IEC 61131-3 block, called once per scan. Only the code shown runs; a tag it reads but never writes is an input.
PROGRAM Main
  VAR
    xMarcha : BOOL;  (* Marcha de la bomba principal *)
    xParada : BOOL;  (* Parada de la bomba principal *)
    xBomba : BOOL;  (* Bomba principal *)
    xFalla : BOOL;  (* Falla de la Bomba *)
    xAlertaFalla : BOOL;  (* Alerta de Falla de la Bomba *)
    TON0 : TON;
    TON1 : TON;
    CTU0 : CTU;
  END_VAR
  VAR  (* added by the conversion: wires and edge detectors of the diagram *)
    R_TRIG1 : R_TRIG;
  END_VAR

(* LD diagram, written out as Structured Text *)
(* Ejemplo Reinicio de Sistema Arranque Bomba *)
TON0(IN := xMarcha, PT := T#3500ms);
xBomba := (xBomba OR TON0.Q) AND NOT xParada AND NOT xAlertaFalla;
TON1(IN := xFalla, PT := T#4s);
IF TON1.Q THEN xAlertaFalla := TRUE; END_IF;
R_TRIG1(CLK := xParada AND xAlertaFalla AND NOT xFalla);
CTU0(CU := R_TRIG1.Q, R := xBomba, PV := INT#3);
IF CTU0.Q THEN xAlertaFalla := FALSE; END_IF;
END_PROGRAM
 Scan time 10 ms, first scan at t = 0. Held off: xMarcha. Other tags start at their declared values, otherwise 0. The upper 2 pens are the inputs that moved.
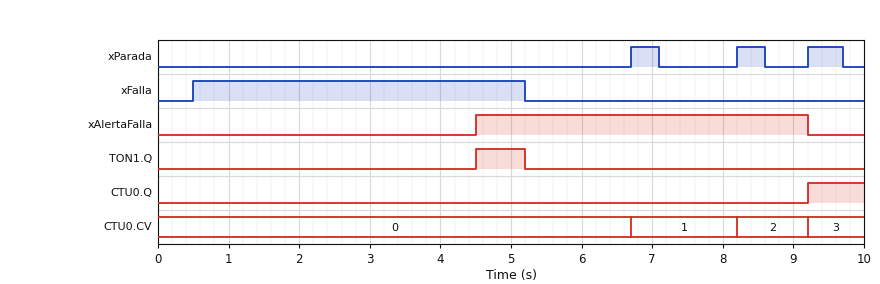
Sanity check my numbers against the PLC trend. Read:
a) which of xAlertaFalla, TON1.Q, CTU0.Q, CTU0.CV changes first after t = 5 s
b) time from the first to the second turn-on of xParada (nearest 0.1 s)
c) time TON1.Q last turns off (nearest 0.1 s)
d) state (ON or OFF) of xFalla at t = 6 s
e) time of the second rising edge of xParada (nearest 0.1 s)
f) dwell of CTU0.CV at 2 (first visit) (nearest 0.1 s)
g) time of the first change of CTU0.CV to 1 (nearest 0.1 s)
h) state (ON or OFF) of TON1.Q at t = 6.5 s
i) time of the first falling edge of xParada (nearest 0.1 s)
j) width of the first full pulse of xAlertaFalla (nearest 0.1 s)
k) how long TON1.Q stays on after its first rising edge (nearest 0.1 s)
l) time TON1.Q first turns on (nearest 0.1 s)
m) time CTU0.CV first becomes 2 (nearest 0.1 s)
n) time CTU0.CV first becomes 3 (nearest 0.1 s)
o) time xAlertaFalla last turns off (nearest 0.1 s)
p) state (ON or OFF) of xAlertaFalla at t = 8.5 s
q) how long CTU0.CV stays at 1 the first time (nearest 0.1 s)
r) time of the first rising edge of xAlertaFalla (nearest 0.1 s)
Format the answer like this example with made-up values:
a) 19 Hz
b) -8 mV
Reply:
a) TON1.Q
b) 1.5 s
c) 5.2 s
d) OFF
e) 8.2 s
f) 1.0 s
g) 6.7 s
h) OFF
i) 7.1 s
j) 4.7 s
k) 0.7 s
l) 4.5 s
m) 8.2 s
n) 9.2 s
o) 9.2 s
p) ON
q) 1.5 s
r) 4.5 s
